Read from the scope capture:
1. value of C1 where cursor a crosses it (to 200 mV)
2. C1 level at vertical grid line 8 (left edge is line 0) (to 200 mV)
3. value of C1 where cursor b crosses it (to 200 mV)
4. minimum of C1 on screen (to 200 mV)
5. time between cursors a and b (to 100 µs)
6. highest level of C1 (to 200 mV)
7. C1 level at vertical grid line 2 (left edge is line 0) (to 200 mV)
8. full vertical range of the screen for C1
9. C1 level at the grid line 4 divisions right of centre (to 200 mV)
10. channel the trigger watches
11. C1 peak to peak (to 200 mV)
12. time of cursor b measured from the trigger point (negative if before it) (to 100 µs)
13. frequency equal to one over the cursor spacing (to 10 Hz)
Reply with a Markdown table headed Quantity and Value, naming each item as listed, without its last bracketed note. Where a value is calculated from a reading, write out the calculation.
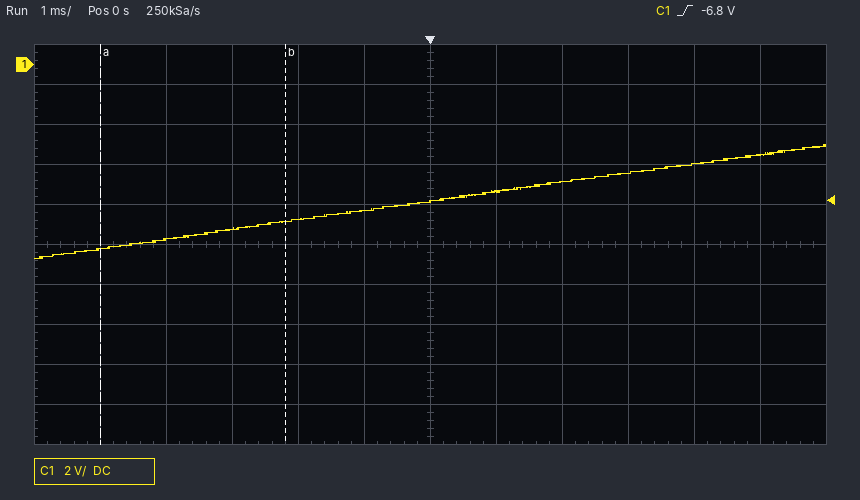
| Quantity | Value |
|---|---|
| value of C1 where cursor a crosses it | -9.2 V |
| C1 level at vertical grid line 8 (left edge is line 0) | -5.8 V |
| value of C1 where cursor b crosses it | -7.8 V |
| minimum of C1 on screen | -9.6 V |
| time between cursors a and b | 2.8 ms |
| highest level of C1 | -4.0 V |
| C1 level at vertical grid line 2 (left edge is line 0) | -8.8 V |
| full vertical range of the screen for C1 | 20 V |
| C1 level at the grid line 4 divisions right of centre | -5.0 V |
| channel the trigger watches | C1 |
| C1 peak to peak | -4.0 V − (-9.6 V) = 5.6 V |
| time of cursor b measured from the trigger point (negative if before it) | -2.2 ms |
| frequency equal to one over the cursor spacing | 1 / 2.8 ms ≈ 360 Hz |
